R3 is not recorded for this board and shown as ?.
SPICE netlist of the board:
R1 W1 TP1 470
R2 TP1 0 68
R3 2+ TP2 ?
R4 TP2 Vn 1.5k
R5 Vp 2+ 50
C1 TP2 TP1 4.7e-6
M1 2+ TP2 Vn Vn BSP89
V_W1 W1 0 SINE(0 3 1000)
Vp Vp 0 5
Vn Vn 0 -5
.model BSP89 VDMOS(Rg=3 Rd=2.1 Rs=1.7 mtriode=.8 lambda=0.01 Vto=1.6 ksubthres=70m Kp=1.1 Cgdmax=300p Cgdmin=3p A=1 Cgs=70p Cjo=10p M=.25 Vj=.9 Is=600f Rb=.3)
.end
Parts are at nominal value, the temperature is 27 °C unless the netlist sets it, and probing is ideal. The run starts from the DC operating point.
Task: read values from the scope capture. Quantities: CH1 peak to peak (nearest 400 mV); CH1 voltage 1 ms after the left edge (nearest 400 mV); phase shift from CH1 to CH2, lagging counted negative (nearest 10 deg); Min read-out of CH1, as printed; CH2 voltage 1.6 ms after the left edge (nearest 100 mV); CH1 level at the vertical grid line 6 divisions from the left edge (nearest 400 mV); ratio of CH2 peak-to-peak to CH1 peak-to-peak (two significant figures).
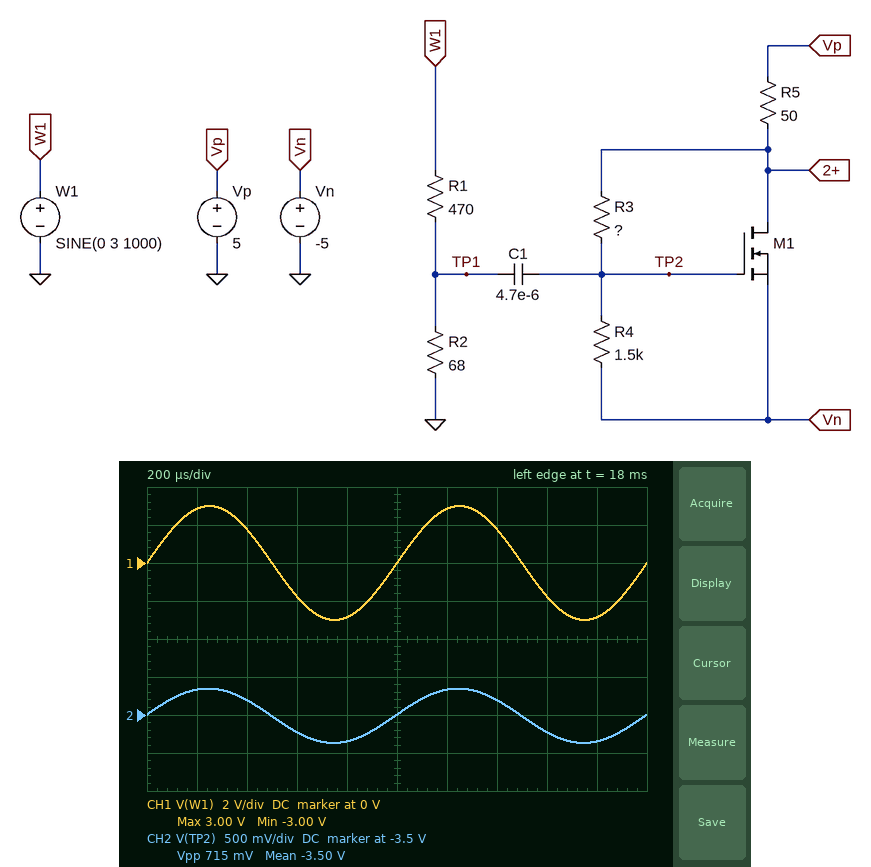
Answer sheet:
6.0 V
0 V
0 deg
-3.00 V
-3.7 V
2.8 V
0.12
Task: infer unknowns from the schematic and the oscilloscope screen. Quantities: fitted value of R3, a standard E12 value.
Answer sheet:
8.2 kΩ
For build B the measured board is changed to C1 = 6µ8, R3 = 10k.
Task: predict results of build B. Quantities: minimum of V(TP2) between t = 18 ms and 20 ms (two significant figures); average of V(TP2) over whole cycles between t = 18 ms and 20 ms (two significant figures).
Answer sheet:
-4.1 V
-3.7 V
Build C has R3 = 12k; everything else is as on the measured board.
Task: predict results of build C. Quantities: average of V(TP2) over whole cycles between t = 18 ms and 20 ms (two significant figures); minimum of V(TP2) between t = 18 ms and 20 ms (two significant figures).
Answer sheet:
-3.9 V
-4.3 V
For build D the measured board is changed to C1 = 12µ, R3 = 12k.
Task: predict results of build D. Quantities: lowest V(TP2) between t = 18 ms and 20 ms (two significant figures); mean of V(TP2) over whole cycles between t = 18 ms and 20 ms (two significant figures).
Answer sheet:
-4.3 V
-3.9 V
